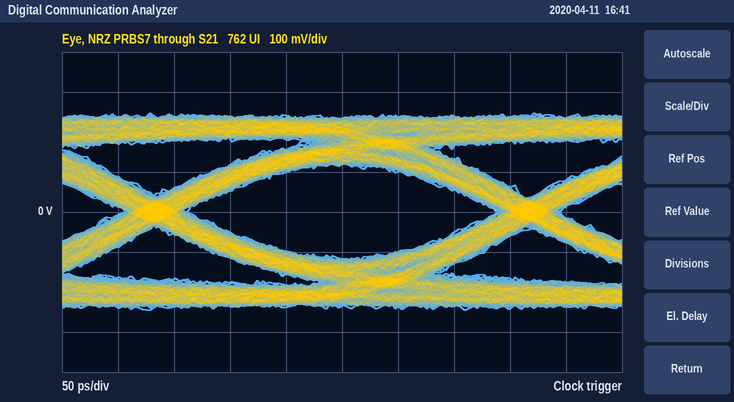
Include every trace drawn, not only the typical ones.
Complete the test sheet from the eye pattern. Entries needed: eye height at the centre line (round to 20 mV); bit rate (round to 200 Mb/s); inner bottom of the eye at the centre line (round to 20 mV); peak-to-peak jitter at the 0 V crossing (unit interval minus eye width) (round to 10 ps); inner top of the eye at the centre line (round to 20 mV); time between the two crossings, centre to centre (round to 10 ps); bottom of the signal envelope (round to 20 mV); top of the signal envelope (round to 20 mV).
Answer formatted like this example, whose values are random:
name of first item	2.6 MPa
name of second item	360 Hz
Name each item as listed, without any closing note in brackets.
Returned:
eye height at the centre line	240 mV
bit rate	3.0 Gb/s
inner bottom of the eye at the centre line	-120 mV
peak-to-peak jitter at the 0 V crossing (unit interval minus eye width)	60 ps
inner top of the eye at the centre line	120 mV
time between the two crossings, centre to centre	330 ps
bottom of the signal envelope	-240 mV
top of the signal envelope	240 mV
